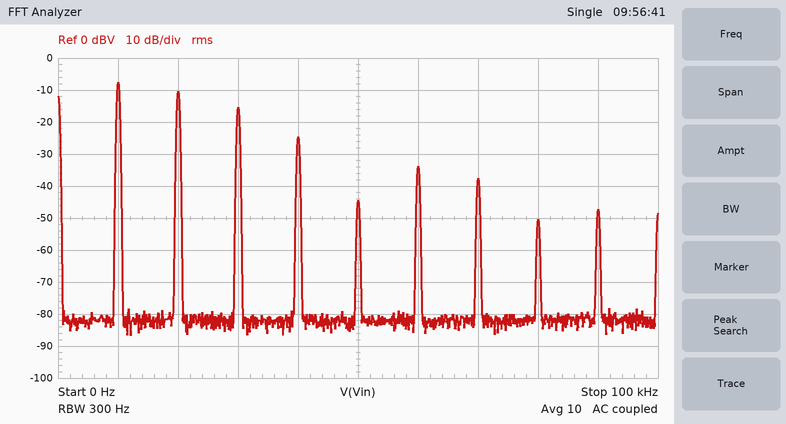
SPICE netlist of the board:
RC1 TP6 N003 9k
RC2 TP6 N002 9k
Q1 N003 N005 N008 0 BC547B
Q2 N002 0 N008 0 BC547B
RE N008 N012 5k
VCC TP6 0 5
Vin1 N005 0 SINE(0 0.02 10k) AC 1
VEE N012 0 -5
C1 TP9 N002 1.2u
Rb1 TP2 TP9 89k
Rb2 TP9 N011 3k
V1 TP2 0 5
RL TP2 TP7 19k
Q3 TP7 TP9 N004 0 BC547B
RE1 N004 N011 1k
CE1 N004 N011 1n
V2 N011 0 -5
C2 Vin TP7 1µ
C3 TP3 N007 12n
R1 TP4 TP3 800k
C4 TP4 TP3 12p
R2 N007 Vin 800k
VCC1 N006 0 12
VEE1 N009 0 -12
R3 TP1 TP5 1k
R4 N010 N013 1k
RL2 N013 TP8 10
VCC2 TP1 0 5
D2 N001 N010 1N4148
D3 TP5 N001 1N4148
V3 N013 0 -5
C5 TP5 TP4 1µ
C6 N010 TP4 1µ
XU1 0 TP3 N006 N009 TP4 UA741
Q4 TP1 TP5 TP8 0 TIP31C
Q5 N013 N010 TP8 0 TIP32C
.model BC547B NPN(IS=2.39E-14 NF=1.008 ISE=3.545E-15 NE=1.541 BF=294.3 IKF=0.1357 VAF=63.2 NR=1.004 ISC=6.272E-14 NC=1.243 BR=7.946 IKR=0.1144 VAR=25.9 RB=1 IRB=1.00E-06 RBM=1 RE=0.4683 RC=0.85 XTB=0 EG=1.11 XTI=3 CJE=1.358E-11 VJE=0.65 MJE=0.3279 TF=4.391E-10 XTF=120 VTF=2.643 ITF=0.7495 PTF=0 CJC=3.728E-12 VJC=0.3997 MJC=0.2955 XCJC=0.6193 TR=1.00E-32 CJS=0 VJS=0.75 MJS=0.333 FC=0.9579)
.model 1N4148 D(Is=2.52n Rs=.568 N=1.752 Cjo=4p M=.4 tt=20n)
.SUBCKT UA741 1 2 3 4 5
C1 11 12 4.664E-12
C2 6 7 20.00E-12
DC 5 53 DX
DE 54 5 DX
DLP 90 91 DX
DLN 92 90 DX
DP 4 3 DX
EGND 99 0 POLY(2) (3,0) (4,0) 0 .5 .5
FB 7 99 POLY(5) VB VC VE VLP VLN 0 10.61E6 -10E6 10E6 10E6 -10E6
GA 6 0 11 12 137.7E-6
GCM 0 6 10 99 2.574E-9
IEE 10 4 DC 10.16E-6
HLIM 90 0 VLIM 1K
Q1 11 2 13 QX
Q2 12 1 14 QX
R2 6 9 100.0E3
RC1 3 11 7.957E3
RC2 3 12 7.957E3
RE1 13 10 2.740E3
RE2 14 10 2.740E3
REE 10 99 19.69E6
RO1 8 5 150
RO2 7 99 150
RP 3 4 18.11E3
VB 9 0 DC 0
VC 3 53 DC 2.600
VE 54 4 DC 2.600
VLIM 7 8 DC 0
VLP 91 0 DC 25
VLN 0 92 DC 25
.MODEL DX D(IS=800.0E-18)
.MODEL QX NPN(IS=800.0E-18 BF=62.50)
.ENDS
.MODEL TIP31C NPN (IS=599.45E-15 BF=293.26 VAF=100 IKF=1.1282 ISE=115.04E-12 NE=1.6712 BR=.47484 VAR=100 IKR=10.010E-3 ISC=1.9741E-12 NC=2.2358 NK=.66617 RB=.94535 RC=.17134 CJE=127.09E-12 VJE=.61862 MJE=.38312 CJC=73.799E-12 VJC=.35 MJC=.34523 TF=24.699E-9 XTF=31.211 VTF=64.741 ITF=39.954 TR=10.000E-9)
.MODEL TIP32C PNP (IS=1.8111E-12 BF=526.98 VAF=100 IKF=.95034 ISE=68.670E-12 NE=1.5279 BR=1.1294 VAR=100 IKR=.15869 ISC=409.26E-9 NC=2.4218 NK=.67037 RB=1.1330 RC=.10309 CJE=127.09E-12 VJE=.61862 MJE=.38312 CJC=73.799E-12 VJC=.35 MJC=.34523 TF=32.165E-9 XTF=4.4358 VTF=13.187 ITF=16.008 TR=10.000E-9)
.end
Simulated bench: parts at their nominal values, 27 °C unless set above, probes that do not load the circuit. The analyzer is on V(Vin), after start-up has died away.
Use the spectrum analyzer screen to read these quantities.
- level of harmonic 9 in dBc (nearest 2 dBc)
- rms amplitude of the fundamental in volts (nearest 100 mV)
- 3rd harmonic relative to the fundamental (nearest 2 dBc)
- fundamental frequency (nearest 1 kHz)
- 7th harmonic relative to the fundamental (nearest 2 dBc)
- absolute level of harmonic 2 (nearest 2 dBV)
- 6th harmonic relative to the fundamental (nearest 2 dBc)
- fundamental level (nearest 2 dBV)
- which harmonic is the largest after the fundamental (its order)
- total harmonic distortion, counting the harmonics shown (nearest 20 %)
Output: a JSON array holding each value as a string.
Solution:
["-40 dBc", "400 mV", "-8 dBc", "10 kHz", "-30 dBc", "-10 dBV", "-26 dBc", "-8 dBV", "2", "80 %"]
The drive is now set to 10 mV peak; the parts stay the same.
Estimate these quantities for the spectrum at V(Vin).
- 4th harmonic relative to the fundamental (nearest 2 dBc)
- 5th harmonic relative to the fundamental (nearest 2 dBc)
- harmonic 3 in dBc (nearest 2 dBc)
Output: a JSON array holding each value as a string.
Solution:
["-12 dBc", "-18 dBc", "-6 dBc"]
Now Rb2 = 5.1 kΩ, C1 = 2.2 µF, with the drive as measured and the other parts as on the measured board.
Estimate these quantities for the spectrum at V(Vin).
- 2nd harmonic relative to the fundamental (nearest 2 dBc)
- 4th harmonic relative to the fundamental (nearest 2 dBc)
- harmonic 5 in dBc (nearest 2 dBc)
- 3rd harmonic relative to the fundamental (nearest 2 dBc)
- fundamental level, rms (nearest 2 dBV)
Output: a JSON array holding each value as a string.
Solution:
["-8 dBc", "-22 dBc", "-40 dBc", "-36 dBc", "8 dBV"]
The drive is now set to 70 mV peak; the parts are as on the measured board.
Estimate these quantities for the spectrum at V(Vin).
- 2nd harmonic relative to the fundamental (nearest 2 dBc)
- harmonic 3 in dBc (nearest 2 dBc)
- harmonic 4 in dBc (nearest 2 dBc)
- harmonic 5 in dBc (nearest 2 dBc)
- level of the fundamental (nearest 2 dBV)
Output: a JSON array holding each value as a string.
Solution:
["-6 dBc", "-32 dBc", "-20 dBc", "-32 dBc", "8 dBV"]
